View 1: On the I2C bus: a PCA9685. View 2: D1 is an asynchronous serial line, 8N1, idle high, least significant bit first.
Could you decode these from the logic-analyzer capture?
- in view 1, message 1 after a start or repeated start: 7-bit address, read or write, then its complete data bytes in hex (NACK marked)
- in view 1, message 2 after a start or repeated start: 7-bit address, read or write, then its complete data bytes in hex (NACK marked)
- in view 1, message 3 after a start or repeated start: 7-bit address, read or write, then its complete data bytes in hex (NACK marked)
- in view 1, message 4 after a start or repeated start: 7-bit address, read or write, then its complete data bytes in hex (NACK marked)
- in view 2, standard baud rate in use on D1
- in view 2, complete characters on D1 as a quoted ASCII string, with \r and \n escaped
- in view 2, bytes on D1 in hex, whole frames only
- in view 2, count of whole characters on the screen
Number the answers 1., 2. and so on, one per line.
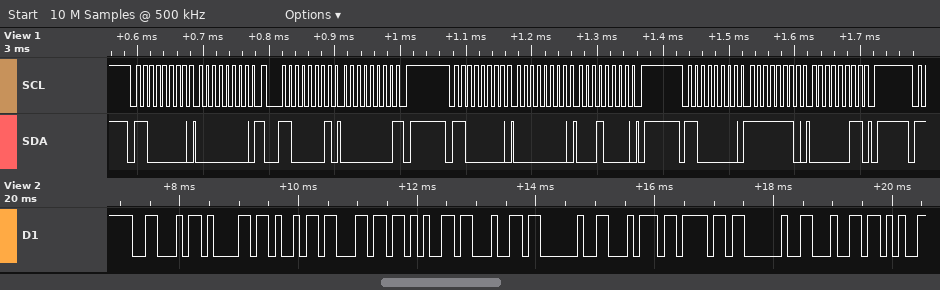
1. 0x60 write: 00
2. 0x60 read: 00 NACK
3. 0x60 write: 00 10
4. 0x60 write: FE 03
5. 9600 baud
6. "Failed to d"
7. 46 61 69 6C 65 64 20 74 6F 20 64
8. 11
